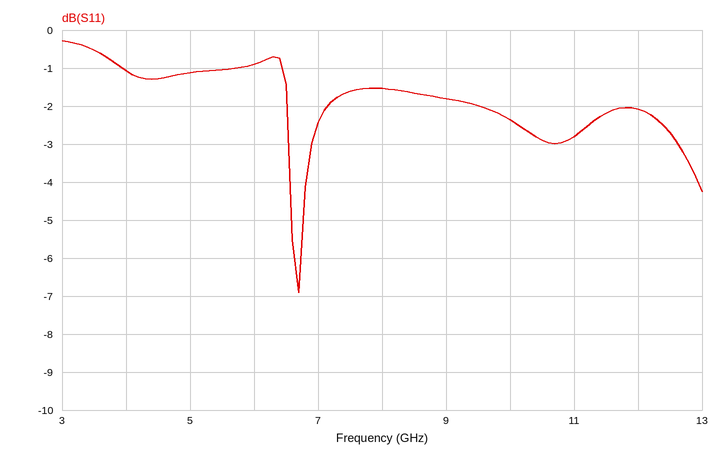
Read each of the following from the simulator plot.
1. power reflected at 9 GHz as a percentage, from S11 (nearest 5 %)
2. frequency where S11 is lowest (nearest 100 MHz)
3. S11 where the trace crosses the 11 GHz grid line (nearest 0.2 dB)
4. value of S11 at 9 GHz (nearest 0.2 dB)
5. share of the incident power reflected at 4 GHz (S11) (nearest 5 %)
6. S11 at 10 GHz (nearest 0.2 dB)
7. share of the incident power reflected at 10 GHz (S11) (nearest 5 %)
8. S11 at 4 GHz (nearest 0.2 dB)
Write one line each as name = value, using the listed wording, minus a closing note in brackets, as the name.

power reflected at 9 GHz as a percentage, from S11 = 65 %
frequency where S11 is lowest = 6.7 GHz
S11 where the trace crosses the 11 GHz grid line = -2.8 dB
value of S11 at 9 GHz = -1.8 dB
share of the incident power reflected at 4 GHz (S11) = 80 %
S11 at 10 GHz = -2.4 dB
share of the incident power reflected at 10 GHz (S11) = 60 %
S11 at 4 GHz = -1.0 dB
